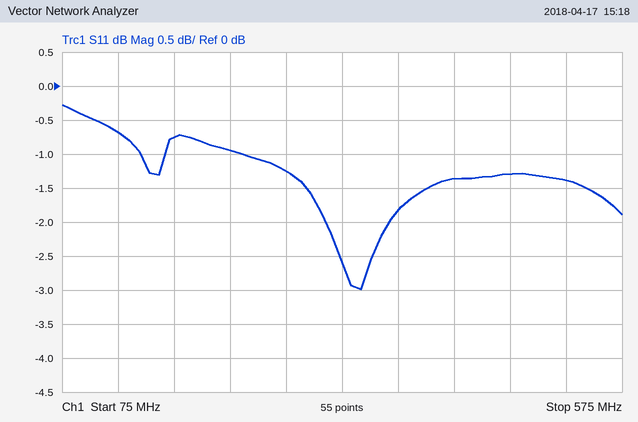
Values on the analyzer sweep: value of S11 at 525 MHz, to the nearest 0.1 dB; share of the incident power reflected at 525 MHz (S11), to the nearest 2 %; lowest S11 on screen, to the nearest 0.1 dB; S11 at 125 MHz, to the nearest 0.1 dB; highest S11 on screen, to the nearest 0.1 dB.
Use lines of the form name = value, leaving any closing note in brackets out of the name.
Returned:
value of S11 at 525 MHz, to the nearest 0.1 dB = -1.4 dB
share of the incident power reflected at 525 MHz (S11), to the nearest 2 % = 72 %
lowest S11 on screen, to the nearest 0.1 dB = -3.0 dB
S11 at 125 MHz, to the nearest 0.1 dB = -0.7 dB
highest S11 on screen, to the nearest 0.1 dB = -0.3 dB
